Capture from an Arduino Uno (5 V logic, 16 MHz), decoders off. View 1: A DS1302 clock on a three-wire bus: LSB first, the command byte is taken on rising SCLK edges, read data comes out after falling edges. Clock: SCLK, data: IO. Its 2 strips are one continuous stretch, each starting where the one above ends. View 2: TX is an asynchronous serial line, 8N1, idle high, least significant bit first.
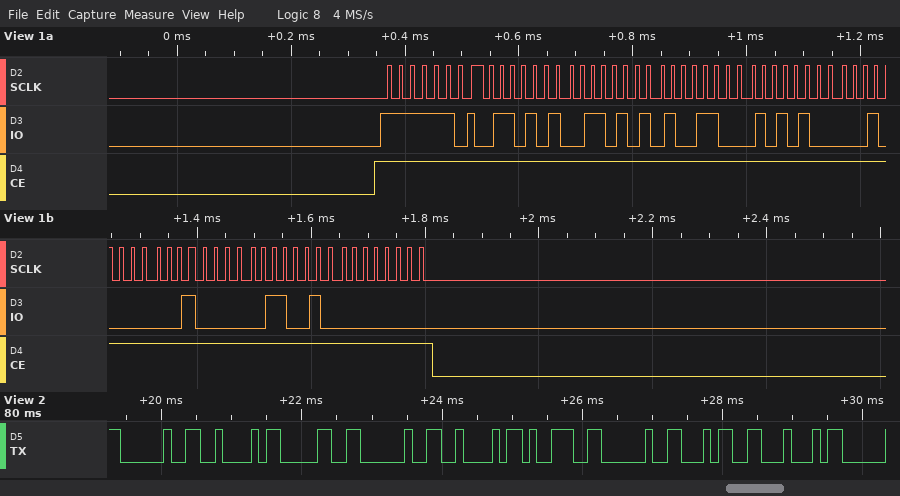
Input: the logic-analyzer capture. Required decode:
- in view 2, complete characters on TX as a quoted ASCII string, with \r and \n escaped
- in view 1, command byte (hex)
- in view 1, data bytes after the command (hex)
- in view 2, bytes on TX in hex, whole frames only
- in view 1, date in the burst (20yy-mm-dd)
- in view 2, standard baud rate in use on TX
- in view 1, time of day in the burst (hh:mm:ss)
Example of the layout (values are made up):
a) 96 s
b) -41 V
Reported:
a) " B0 B9 4D"
b) 0xBF
c) 56 56 19 15 04 04 26 00
d) 20 42 30 20 42 39 20 34 44
e) 2026-04-15
f) 9600 baud
g) 19:56:56
